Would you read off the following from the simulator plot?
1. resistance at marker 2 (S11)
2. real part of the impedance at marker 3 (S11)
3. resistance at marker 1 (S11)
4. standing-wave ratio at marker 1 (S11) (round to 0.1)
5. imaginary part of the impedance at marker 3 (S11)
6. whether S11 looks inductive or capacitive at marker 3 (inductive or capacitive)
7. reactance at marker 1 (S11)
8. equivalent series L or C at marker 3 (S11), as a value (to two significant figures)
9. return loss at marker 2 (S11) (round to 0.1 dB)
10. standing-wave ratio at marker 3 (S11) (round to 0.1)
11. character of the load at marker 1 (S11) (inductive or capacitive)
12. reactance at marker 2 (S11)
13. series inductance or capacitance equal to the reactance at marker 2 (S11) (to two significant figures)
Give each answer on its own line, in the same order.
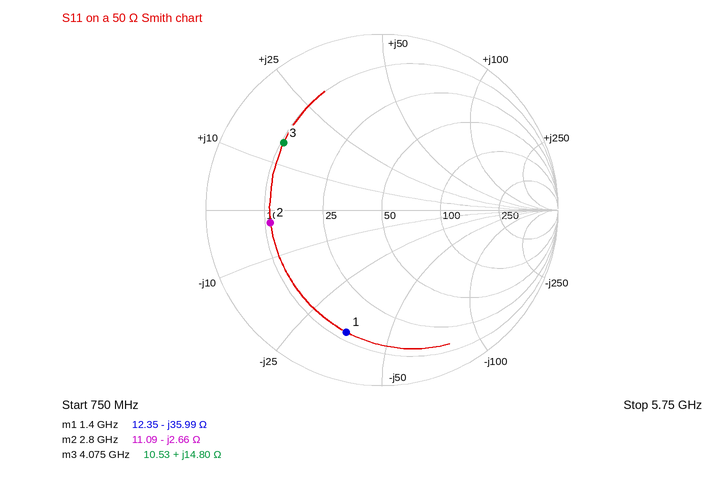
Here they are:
11.09 Ω
10.53 Ω
12.35 Ω
6.2
+14.80 Ω
inductive
-35.99 Ω
580 pH
3.9 dB
5.2
capacitive
-2.66 Ω
21 pF
